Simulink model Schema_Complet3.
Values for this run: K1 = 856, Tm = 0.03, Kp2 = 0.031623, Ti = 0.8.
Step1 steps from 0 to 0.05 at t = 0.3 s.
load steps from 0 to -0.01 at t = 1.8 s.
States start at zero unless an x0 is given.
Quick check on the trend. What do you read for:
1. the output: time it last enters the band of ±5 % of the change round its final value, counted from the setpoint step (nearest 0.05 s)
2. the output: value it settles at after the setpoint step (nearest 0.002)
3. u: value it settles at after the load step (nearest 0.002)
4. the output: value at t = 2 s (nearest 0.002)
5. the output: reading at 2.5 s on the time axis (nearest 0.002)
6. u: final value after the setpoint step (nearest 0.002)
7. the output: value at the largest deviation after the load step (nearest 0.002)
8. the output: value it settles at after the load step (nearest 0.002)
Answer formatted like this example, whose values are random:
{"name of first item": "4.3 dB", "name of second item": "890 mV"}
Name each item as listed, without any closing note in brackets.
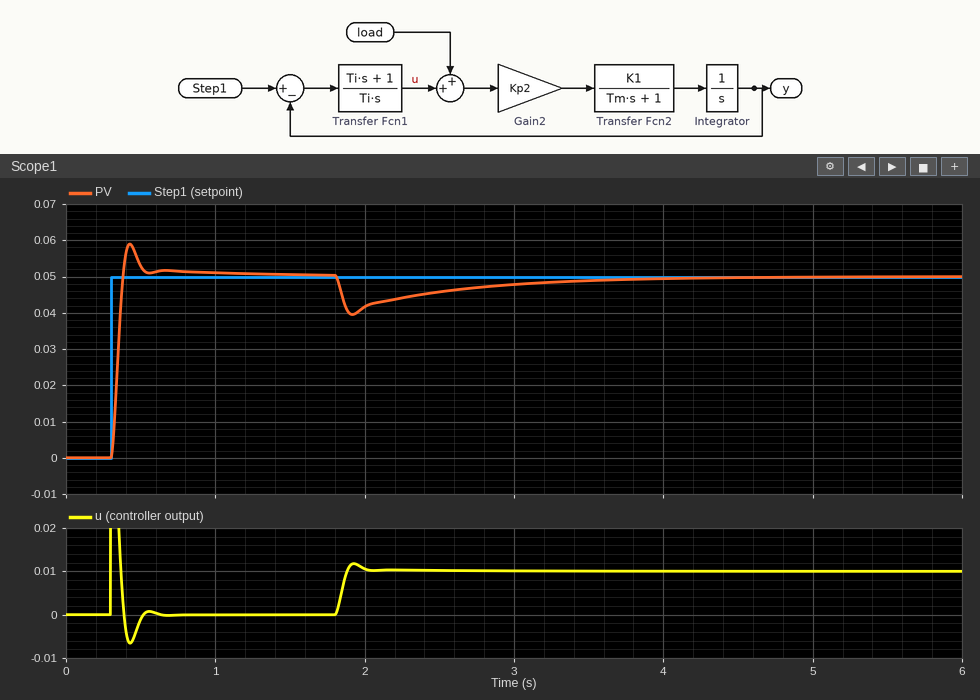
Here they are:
{"the output: time it last enters the band of ±5 % of the change round its final value, counted from the setpoint step": "0.20 s", "the output: value it settles at after the setpoint step": "0.050", "u: value it settles at after the load step": "0.010", "the output: value at t = 2 s": "0.042", "the output: reading at 2.5 s on the time axis": "0.046", "u: final value after the setpoint step": "0.000", "the output: value at the largest deviation after the load step": "0.040", "the output: value it settles at after the load step": "0.050"}
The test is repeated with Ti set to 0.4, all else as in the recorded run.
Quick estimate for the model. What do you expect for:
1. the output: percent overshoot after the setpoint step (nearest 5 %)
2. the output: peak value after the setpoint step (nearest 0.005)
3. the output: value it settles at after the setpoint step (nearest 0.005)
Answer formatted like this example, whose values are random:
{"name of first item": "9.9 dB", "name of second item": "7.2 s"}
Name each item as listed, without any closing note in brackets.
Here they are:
{"the output: percent overshoot after the setpoint step": "25 %", "the output: peak value after the setpoint step": "0.060", "the output: value it settles at after the setpoint step": "0.050"}
